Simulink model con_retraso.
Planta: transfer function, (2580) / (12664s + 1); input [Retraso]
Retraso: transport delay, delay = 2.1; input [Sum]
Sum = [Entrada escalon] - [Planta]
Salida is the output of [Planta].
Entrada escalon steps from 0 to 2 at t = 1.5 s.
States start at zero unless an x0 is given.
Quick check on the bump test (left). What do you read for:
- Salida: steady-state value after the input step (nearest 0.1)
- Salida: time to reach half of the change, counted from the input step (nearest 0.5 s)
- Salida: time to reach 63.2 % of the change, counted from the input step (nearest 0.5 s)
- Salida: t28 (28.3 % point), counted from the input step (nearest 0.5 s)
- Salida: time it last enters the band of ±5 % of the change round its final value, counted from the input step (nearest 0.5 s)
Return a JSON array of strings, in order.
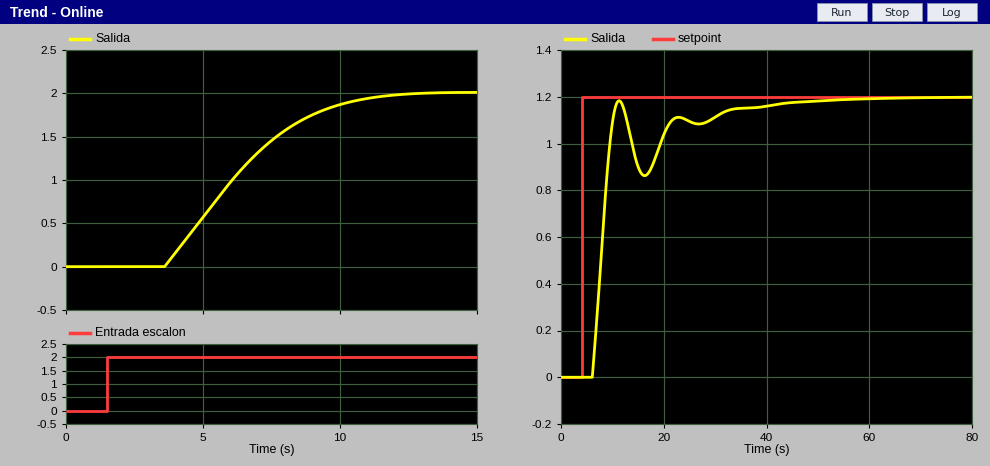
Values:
["2.0", "4.5 s", "5.5 s", "3.5 s", "9.0 s"]
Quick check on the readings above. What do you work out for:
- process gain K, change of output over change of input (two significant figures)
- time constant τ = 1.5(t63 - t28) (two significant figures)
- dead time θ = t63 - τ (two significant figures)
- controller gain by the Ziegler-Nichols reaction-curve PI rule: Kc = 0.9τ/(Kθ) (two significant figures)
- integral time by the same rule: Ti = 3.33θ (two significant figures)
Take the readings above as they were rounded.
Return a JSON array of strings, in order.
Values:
["1.0", "3.0 s", "2.5 s", "1.1", "8.3 s"]
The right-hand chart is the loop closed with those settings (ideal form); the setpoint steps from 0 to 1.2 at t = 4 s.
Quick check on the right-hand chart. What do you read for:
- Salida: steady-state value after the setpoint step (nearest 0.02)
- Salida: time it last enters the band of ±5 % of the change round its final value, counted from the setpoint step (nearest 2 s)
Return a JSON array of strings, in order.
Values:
["1.20", "28 s"]
